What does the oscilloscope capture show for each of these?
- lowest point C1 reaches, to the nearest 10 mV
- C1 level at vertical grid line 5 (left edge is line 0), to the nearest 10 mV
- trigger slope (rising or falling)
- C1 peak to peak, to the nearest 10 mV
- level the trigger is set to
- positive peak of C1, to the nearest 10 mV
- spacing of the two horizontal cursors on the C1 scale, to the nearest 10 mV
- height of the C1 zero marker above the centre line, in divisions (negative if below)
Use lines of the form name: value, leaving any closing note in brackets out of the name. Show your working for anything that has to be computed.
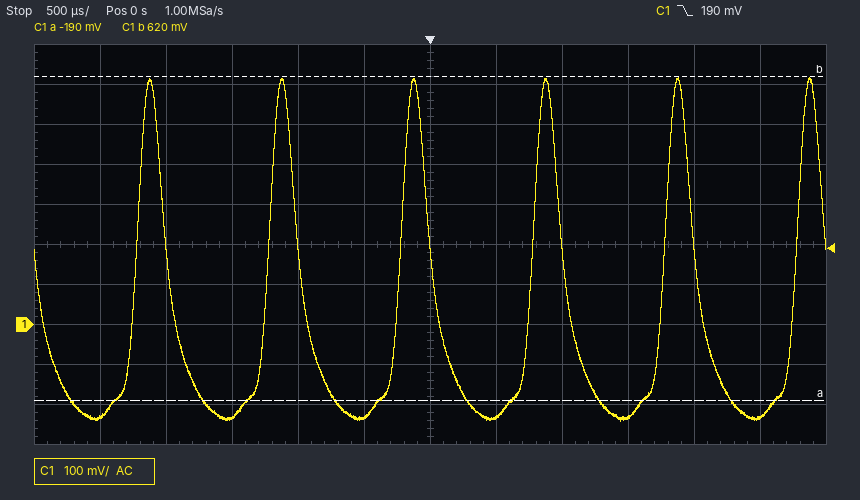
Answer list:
lowest point C1 reaches, to the nearest 10 mV: -240 mV
C1 level at vertical grid line 5 (left edge is line 0), to the nearest 10 mV: -230 mV
trigger slope: falling
C1 peak to peak, to the nearest 10 mV: 620 mV − (-240 mV) = 860 mV
level the trigger is set to: 190 mV
positive peak of C1, to the nearest 10 mV: 620 mV
spacing of the two horizontal cursors on the C1 scale, to the nearest 10 mV: 810 mV
height of the C1 zero marker above the centre line, in divisions: -2.0 div
